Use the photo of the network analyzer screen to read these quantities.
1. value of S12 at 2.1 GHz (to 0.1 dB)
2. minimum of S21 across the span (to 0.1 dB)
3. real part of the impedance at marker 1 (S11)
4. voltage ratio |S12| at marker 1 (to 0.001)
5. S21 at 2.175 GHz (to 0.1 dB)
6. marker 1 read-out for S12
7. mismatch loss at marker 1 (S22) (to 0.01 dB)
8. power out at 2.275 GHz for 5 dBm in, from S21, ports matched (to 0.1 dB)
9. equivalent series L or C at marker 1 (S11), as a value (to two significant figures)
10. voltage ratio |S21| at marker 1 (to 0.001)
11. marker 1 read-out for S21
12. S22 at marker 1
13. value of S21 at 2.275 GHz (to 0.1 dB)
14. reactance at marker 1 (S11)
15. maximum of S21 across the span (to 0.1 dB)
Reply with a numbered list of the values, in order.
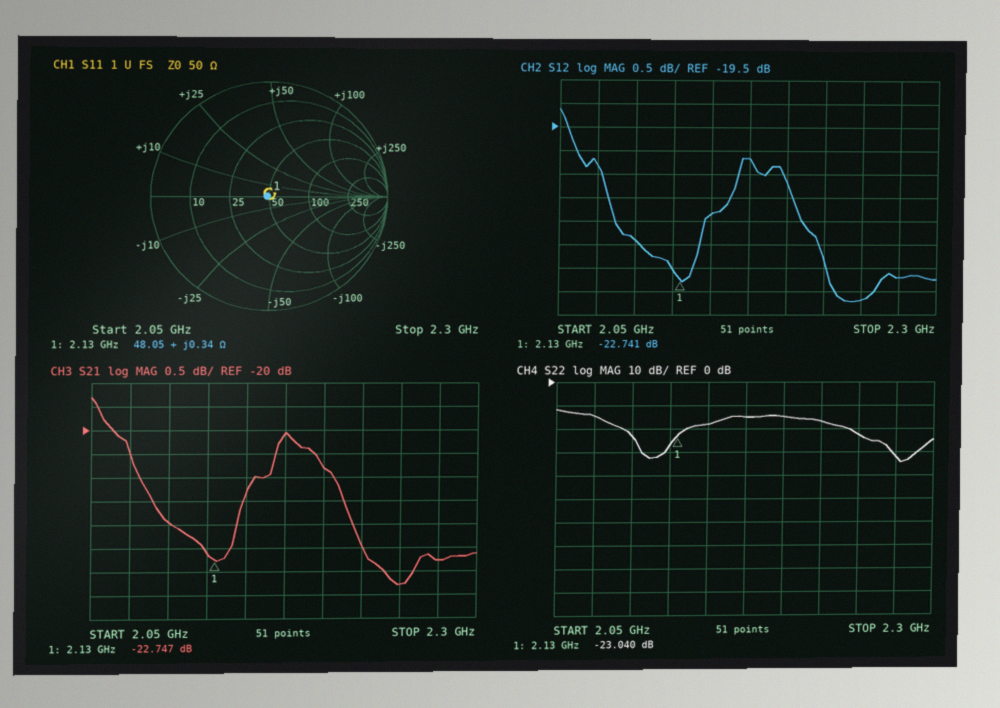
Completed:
1. -21.9 dB
2. -23.3 dB
3. 48.05 Ω
4. 0.073
5. -20.1 dB
6. -22.741 dB
7. 0.02 dB
8. -17.8 dBm
9. 25 pH
10. 0.073
11. -22.747 dB
12. -23.040 dB
13. -22.8 dB
14. +0.34 Ω
15. -19.3 dB
